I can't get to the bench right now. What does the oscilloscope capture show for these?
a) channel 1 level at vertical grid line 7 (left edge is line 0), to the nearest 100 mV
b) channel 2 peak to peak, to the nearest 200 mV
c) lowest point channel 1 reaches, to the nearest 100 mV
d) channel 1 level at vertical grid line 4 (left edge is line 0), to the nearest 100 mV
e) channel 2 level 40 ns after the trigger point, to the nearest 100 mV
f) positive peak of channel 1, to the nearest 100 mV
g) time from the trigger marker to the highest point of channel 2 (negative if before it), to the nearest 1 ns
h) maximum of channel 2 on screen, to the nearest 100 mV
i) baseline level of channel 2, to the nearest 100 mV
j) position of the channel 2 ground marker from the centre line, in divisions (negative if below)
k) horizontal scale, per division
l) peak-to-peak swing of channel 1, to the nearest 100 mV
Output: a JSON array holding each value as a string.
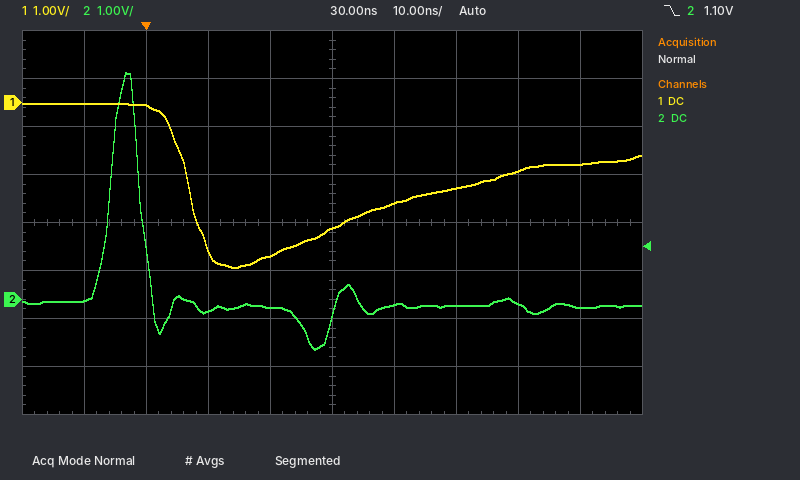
["-1.8 V", "5.8 V", "-3.4 V", "-3.2 V", "-100 mV", "0.0 V", "-3 ns", "4.7 V", "-100 mV", "-1.6 div", "10 ns", "3.4 V"]
